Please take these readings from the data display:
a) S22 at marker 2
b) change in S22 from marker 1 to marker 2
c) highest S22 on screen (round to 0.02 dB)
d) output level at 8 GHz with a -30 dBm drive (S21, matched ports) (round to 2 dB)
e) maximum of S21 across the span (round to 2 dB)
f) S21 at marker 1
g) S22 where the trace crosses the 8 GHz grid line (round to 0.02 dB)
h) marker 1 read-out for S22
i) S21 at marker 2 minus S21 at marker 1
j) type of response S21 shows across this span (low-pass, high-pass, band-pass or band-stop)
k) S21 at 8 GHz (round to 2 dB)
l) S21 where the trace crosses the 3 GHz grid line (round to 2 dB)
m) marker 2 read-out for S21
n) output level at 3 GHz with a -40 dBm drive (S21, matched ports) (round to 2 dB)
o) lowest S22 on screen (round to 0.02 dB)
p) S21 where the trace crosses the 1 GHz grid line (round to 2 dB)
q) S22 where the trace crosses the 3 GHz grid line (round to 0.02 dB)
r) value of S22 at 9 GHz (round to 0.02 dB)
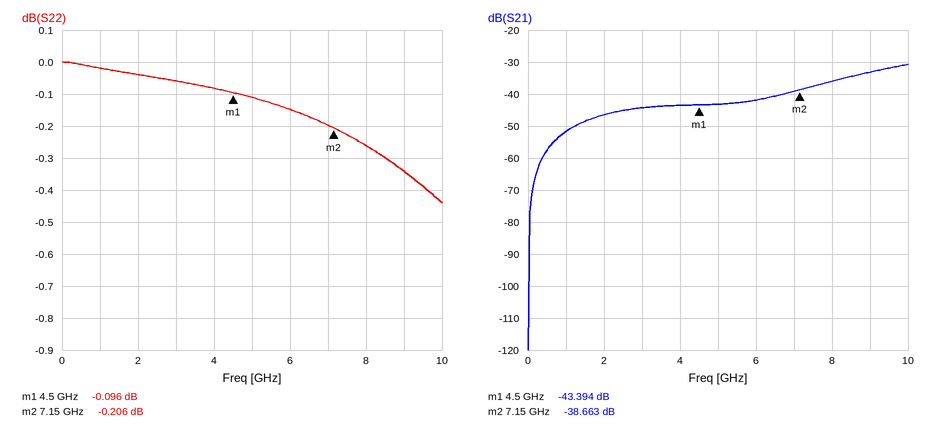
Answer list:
-0.206 dB
-0.110 dB
0.00 dB
-66 dBm
-30 dB
-43.394 dB
-0.26 dB
-0.096 dB
4.731 dB
high-pass
-36 dB
-44 dB
-38.663 dB
-84 dBm
-0.44 dB
-52 dB
-0.06 dB
-0.34 dB
